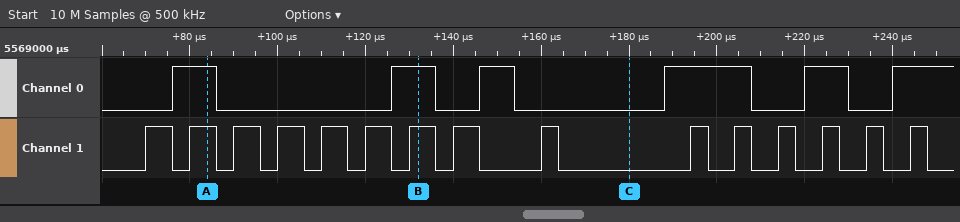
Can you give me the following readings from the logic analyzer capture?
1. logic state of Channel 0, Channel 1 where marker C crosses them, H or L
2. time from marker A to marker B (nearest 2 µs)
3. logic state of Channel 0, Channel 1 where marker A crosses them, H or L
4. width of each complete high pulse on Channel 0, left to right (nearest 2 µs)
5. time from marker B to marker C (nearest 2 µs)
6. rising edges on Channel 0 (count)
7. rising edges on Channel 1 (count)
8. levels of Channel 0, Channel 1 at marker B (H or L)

Channel 0=L, Channel 1=L
48 µs
Channel 0=H, Channel 1=H
10 µs, 10 µs, 8 µs, 20 µs, 10 µs
48 µs
6
15
Channel 0=H, Channel 1=H
